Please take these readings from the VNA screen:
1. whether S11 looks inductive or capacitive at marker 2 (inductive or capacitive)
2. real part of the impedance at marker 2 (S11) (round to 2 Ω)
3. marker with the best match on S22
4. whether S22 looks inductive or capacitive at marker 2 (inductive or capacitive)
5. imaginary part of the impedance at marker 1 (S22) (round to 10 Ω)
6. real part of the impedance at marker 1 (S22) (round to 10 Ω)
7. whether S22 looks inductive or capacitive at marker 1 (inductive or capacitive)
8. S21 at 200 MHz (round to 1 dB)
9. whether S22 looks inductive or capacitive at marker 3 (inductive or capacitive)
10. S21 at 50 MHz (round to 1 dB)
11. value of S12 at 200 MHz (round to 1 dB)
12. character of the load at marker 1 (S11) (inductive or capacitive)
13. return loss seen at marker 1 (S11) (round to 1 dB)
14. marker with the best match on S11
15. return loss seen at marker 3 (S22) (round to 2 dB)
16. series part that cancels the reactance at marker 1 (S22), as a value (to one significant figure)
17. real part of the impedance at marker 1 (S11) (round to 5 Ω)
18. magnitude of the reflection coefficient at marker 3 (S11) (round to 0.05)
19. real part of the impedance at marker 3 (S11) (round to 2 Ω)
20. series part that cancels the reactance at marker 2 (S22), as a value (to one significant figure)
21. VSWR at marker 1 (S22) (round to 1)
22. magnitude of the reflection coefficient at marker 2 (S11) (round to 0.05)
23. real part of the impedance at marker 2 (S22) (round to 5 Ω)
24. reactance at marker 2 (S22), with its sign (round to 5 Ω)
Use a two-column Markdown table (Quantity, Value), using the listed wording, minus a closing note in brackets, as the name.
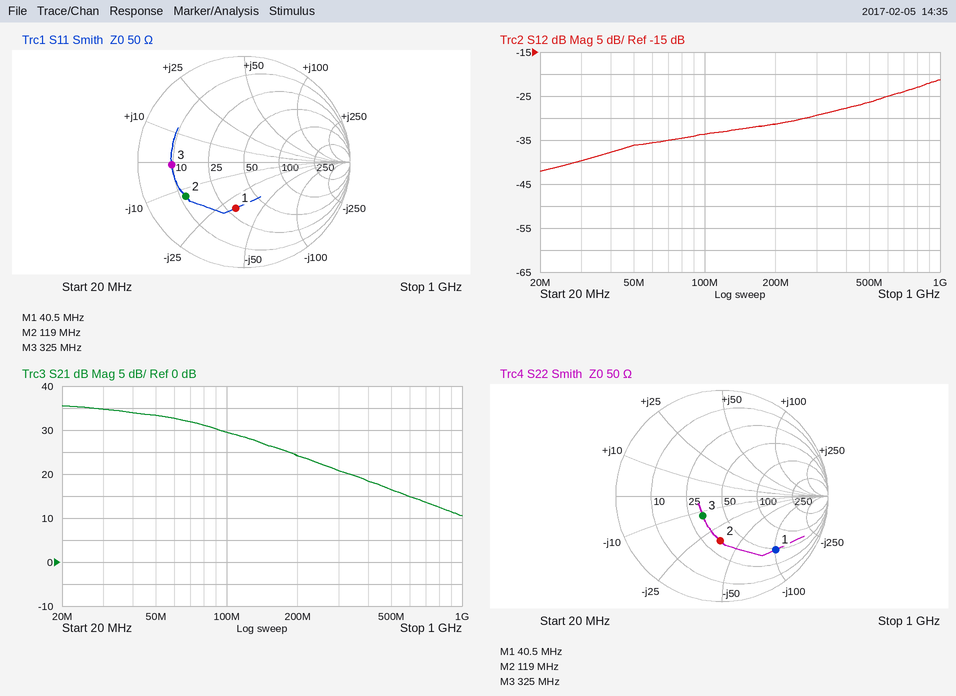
| Quantity | Value |
|---|---|
| whether S11 looks inductive or capacitive at marker 2 | capacitive |
| real part of the impedance at marker 2 (S11) | 12 Ω |
| marker with the best match on S22 | marker 3 |
| whether S22 looks inductive or capacitive at marker 2 | capacitive |
| imaginary part of the impedance at marker 1 (S22) | -100 Ω |
| real part of the impedance at marker 1 (S22) | 50 Ω |
| whether S22 looks inductive or capacitive at marker 1 | capacitive |
| S21 at 200 MHz | 24 dB |
| whether S22 looks inductive or capacitive at marker 3 | capacitive |
| S21 at 50 MHz | 33 dB |
| value of S12 at 200 MHz | -31 dB |
| character of the load at marker 1 (S11) | capacitive |
| return loss seen at marker 1 (S11) | 7 dB |
| marker with the best match on S11 | marker 1 |
| return loss seen at marker 3 (S22) | 12 dB |
| series part that cancels the reactance at marker 1 (S22), as a value | 400 nH |
| real part of the impedance at marker 1 (S11) | 30 Ω |
| magnitude of the reflection coefficient at marker 3 (S11) | 0.70 |
| real part of the impedance at marker 3 (S11) | 10 Ω |
| series part that cancels the reactance at marker 2 (S22), as a value | 50 nH |
| VSWR at marker 1 (S22) | 6 |
| magnitude of the reflection coefficient at marker 2 (S11) | 0.65 |
| real part of the impedance at marker 2 (S22) | 35 Ω |
| reactance at marker 2 (S22), with its sign | -35 Ω |
